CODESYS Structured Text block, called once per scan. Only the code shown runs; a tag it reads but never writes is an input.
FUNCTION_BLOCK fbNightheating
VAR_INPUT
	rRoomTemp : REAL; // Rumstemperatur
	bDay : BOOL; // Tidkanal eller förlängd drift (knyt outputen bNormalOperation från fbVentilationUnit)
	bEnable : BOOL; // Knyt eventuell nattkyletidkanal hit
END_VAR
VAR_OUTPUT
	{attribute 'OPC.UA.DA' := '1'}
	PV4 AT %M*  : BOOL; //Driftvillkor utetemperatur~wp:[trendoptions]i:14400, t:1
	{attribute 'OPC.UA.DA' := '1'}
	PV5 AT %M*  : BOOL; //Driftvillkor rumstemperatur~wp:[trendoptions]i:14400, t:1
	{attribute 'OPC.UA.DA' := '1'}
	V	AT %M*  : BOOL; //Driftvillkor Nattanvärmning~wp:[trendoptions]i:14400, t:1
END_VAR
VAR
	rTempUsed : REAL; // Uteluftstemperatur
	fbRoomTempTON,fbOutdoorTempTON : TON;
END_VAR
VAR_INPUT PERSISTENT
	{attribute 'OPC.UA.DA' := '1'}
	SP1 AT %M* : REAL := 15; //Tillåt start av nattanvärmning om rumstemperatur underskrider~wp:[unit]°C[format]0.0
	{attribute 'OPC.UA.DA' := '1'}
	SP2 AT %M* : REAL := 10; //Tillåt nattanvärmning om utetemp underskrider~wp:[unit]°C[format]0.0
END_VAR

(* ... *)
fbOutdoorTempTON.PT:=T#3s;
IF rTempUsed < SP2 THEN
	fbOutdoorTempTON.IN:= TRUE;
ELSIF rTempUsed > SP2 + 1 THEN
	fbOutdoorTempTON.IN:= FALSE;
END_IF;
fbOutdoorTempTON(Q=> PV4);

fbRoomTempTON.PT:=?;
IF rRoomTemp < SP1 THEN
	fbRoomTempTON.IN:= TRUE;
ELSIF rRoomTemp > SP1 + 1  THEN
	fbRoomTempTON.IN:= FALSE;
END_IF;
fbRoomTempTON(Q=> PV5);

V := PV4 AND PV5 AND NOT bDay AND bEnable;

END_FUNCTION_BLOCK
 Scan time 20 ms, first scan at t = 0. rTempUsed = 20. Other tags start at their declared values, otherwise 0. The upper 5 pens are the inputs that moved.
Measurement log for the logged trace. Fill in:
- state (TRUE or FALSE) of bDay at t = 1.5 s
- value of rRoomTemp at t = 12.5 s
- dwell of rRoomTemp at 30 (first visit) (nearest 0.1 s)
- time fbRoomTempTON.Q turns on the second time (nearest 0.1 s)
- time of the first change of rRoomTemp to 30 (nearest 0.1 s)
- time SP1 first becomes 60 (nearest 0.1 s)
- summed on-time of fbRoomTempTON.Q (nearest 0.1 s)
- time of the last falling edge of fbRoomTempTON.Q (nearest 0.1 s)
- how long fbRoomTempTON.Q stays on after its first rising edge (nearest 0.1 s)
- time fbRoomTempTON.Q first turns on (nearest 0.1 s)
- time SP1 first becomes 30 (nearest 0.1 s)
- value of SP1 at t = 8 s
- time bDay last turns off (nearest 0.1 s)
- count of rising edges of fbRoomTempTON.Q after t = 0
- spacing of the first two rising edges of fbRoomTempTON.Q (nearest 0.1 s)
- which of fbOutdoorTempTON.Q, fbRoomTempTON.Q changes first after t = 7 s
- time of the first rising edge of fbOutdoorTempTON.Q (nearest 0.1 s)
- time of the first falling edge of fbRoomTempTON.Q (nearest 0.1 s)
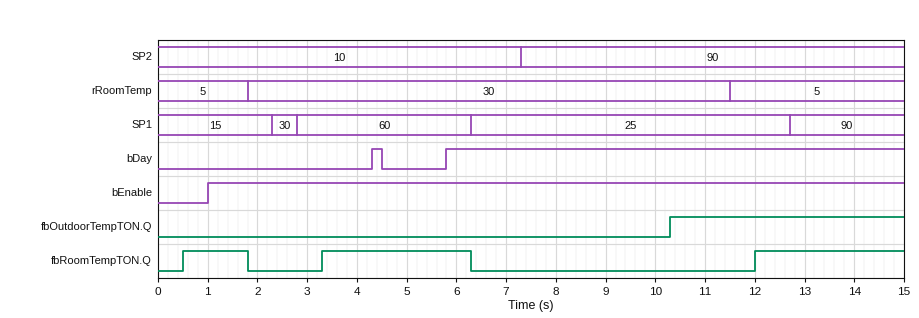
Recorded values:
FALSE
5
9.7 s
3.3 s
1.8 s
2.8 s
7.3 s
6.3 s
1.3 s
0.5 s
2.3 s
25
4.5 s
3
2.8 s
fbOutdoorTempTON.Q
10.3 s
1.8 s
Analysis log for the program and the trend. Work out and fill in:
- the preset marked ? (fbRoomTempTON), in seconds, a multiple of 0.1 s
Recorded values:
0.5 s
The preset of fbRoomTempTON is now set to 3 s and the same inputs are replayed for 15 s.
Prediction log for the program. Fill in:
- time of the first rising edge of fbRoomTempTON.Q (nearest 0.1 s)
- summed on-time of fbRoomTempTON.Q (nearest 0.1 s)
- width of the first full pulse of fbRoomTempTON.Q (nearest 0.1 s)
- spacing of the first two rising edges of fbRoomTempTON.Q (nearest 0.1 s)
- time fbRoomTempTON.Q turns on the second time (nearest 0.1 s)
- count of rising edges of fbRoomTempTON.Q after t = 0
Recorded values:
5.8 s
1.0 s
0.5 s
8.7 s
14.5 s
2
